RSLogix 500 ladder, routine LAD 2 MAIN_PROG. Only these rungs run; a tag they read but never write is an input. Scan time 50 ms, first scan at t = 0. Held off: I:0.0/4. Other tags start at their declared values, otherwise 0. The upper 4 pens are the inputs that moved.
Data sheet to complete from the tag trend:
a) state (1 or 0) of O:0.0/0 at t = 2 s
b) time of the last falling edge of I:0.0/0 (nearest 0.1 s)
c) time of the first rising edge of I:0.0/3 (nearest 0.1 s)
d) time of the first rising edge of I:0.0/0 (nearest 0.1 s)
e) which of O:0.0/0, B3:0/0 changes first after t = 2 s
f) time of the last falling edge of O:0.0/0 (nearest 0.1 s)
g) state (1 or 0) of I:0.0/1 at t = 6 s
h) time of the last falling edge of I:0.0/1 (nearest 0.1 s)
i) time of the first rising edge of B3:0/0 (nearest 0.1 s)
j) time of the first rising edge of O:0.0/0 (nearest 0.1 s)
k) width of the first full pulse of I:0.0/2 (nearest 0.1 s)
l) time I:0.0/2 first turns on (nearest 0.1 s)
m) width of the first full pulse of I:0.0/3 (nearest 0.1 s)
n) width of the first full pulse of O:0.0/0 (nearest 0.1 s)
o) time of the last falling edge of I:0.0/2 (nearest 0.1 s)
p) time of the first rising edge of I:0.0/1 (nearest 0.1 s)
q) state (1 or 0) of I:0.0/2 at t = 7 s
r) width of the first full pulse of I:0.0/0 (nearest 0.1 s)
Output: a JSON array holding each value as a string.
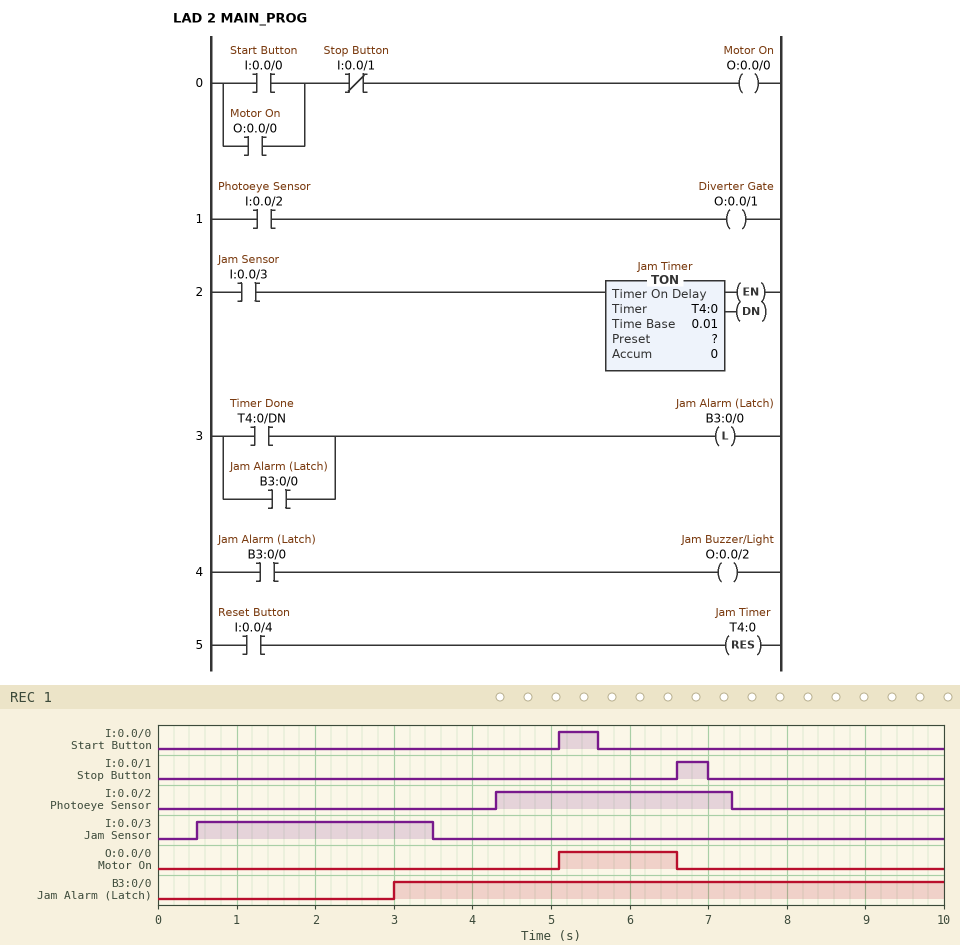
["0", "5.6 s", "0.5 s", "5.1 s", "B3:0/0", "6.6 s", "0", "7.0 s", "3.0 s", "5.1 s", "3.0 s", "4.3 s", "3.0 s", "1.5 s", "7.3 s", "6.6 s", "1", "0.5 s"]
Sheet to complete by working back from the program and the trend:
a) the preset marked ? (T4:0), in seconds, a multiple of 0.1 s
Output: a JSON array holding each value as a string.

["2.5 s"]
